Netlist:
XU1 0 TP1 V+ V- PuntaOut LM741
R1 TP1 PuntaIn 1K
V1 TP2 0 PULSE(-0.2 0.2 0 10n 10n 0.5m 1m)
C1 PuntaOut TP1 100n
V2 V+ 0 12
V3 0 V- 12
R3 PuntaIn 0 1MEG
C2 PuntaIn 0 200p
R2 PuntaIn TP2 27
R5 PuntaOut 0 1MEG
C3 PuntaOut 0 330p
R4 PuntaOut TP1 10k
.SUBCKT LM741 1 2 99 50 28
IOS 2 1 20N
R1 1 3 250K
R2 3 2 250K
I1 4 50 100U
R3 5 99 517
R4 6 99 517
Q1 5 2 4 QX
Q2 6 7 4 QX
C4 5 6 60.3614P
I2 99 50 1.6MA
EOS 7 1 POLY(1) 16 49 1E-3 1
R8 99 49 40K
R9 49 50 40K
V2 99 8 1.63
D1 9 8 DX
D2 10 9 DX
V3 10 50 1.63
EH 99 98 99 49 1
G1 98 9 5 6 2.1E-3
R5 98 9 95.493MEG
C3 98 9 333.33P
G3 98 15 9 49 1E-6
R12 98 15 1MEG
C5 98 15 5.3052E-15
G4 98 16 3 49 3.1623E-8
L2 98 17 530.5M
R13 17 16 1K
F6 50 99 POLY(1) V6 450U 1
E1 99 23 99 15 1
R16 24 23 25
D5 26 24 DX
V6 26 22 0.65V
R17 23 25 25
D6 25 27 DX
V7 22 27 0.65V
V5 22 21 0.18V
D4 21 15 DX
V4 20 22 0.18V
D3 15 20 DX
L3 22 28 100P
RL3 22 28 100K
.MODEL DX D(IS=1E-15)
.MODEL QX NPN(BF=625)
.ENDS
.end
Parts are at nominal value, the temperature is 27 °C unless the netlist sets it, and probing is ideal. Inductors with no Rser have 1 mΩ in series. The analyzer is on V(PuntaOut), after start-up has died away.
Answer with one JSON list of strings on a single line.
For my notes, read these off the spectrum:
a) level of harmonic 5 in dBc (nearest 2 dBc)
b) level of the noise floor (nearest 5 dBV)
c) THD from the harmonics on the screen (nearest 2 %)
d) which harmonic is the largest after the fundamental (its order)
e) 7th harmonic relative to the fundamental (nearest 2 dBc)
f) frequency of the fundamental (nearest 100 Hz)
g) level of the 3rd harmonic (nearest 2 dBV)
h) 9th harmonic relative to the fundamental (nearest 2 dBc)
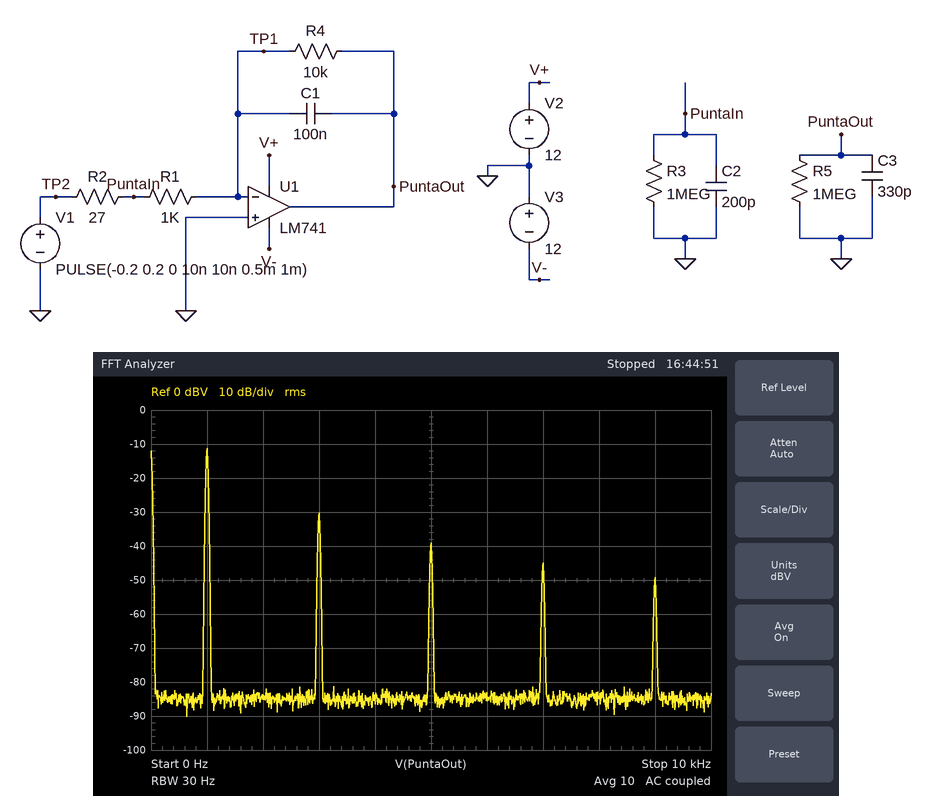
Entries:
["-28 dBc", "-85 dBV", "12 %", "3", "-34 dBc", "1.0 kHz", "-30 dBV", "-38 dBc"]
